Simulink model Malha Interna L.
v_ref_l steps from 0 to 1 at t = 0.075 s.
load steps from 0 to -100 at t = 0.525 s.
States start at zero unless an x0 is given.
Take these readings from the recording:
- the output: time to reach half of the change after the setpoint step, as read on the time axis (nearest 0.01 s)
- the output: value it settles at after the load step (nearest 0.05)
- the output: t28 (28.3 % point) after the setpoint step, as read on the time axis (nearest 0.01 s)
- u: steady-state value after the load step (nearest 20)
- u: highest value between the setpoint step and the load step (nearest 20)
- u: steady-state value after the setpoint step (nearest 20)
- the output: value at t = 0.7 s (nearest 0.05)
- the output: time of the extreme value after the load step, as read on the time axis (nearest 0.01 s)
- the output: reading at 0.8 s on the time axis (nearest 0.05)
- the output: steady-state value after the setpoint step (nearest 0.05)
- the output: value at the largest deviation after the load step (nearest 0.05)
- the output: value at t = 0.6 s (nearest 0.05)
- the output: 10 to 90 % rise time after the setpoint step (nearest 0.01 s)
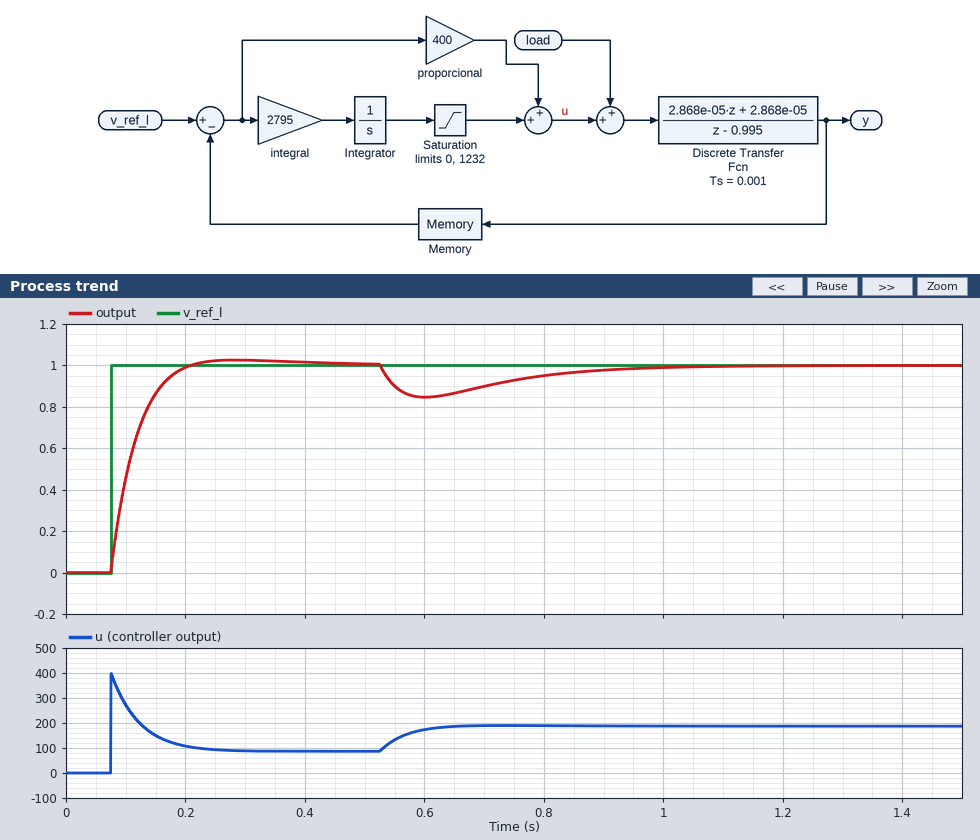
0.10 s
1.00
0.09 s
180
400
80
0.90
0.60 s
0.95
1.00
0.85
0.85
0.08 s
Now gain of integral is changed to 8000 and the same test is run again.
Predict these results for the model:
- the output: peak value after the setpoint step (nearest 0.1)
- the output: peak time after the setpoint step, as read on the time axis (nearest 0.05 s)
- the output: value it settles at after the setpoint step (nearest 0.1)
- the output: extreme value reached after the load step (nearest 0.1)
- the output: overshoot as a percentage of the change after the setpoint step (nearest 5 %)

1.2
0.20 s
1.0
0.9
15 %
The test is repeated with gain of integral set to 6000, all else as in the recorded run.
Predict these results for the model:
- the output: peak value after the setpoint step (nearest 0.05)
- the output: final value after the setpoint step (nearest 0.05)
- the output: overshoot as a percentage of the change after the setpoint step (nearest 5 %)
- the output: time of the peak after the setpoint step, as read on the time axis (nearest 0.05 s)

1.10
1.00
10 %
0.20 s
